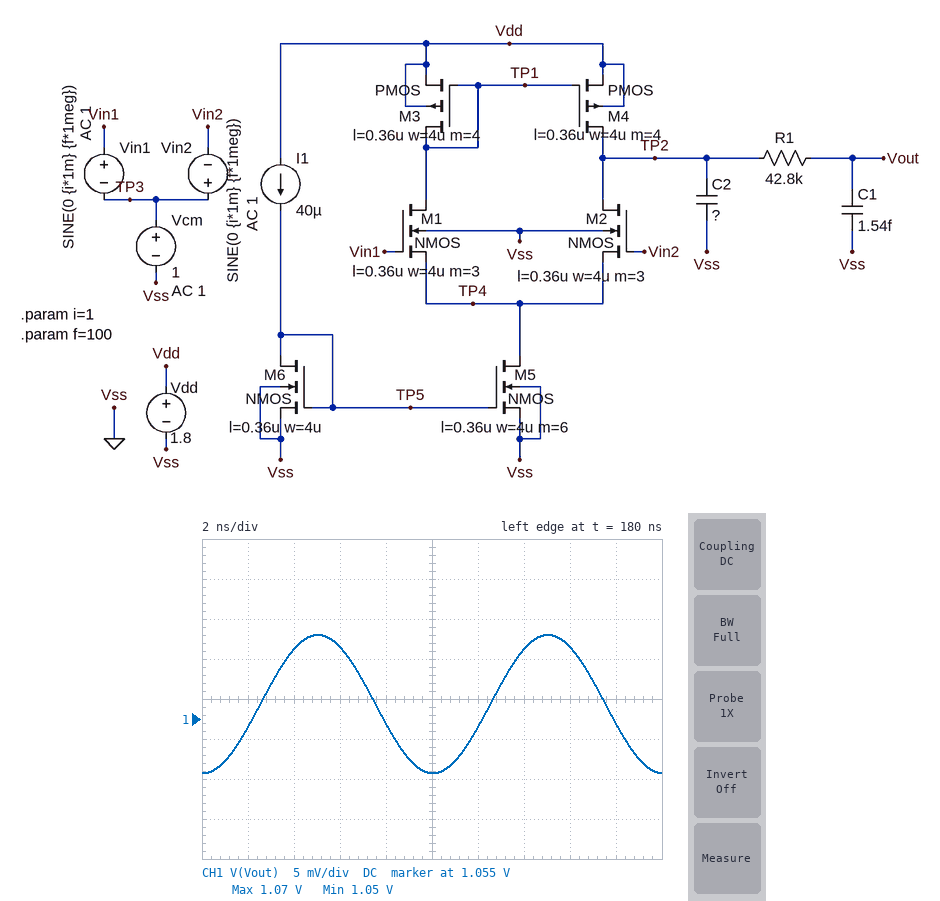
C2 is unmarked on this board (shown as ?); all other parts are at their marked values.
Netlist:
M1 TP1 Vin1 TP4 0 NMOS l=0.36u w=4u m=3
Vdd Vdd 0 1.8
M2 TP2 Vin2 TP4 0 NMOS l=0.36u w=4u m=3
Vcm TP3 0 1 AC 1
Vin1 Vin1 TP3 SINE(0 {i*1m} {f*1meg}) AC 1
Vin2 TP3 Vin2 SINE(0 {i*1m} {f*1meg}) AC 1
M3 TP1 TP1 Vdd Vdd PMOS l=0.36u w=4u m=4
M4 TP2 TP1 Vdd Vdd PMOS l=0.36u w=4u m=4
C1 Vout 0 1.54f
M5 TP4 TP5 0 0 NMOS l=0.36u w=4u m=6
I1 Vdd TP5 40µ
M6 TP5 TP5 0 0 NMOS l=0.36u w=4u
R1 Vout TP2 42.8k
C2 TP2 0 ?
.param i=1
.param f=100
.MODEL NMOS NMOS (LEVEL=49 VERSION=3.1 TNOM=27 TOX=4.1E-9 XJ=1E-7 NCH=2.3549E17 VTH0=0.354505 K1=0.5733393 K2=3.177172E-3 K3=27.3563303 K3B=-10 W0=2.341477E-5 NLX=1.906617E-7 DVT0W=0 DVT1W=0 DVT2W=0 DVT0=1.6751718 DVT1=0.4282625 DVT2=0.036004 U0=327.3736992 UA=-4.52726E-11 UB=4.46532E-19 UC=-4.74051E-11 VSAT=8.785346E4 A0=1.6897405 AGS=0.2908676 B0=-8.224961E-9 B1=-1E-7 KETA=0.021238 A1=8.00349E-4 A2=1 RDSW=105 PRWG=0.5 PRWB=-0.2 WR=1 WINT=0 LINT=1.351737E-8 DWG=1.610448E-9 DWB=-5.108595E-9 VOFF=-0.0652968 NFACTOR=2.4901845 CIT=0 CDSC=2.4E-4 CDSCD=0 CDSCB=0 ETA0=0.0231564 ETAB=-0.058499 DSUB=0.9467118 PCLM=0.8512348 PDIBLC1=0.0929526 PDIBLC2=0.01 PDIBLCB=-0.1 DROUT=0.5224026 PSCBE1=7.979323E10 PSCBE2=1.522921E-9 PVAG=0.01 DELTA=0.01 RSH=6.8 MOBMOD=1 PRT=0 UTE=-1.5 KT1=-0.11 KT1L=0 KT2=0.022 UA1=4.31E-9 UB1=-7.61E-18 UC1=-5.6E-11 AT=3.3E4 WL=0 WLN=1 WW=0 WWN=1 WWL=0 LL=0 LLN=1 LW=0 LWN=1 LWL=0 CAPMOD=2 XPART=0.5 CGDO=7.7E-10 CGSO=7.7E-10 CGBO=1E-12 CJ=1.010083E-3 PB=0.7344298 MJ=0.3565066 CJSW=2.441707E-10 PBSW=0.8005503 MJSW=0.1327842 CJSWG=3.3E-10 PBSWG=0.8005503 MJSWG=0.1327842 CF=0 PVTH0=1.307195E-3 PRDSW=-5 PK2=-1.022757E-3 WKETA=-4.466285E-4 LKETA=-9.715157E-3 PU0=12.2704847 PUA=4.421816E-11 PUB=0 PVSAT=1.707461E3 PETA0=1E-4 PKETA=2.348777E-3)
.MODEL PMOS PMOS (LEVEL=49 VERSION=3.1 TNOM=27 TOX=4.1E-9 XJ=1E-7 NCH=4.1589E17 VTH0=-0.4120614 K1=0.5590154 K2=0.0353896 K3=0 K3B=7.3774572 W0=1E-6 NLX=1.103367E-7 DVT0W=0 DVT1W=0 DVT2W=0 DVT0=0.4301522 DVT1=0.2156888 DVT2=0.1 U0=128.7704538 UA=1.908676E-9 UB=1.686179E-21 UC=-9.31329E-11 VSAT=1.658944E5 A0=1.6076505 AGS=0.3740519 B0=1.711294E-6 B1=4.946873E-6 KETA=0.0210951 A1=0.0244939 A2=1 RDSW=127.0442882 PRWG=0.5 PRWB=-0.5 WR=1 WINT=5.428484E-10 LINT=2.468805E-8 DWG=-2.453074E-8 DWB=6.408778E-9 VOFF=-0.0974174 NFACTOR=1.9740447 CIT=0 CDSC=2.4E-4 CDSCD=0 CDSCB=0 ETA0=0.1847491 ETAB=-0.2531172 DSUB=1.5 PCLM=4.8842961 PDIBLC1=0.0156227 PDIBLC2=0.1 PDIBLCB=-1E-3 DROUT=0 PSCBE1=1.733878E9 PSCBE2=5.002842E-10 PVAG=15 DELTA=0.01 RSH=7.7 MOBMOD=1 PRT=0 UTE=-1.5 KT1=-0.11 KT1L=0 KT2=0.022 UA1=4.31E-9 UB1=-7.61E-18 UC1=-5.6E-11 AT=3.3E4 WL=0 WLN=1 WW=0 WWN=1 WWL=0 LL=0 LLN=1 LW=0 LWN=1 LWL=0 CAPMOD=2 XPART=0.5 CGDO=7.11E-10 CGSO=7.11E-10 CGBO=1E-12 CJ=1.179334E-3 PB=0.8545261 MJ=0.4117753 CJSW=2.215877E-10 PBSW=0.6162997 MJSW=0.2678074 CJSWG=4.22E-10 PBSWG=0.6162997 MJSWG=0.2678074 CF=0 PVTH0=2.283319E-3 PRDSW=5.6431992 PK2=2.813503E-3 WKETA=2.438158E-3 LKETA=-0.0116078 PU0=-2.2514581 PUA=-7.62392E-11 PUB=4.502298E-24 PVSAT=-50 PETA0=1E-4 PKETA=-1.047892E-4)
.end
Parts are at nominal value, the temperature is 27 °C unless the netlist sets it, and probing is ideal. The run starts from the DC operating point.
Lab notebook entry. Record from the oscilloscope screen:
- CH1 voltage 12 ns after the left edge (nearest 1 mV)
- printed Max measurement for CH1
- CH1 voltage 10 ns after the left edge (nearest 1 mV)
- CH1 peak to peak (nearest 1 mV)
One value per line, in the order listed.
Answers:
1.054 V
1.07 V
1.048 V
17 mV
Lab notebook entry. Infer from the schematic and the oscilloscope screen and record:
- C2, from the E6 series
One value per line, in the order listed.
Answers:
470 fF
